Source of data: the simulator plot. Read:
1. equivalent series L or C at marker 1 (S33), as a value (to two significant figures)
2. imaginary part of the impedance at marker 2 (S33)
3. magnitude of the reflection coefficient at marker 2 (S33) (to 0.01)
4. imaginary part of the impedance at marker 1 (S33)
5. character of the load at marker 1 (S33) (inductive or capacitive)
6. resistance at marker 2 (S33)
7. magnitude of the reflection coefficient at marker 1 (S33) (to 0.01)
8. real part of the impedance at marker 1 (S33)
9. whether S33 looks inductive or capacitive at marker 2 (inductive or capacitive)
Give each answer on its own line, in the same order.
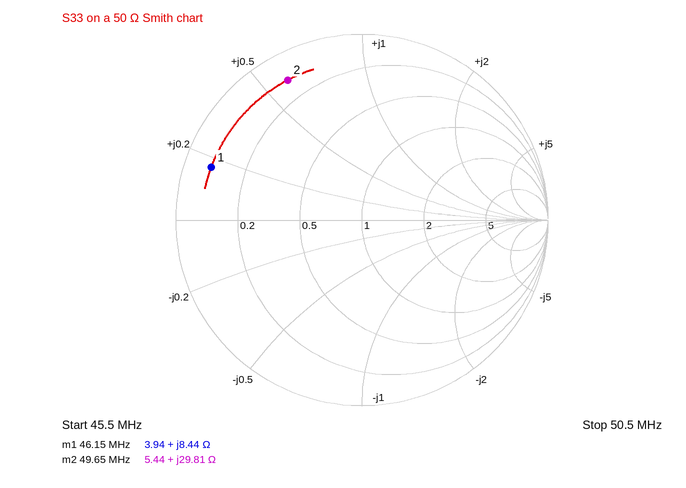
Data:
29 nH
+29.81 Ω
0.85
+8.44 Ω
inductive
5.44 Ω
0.86
3.94 Ω
inductive
